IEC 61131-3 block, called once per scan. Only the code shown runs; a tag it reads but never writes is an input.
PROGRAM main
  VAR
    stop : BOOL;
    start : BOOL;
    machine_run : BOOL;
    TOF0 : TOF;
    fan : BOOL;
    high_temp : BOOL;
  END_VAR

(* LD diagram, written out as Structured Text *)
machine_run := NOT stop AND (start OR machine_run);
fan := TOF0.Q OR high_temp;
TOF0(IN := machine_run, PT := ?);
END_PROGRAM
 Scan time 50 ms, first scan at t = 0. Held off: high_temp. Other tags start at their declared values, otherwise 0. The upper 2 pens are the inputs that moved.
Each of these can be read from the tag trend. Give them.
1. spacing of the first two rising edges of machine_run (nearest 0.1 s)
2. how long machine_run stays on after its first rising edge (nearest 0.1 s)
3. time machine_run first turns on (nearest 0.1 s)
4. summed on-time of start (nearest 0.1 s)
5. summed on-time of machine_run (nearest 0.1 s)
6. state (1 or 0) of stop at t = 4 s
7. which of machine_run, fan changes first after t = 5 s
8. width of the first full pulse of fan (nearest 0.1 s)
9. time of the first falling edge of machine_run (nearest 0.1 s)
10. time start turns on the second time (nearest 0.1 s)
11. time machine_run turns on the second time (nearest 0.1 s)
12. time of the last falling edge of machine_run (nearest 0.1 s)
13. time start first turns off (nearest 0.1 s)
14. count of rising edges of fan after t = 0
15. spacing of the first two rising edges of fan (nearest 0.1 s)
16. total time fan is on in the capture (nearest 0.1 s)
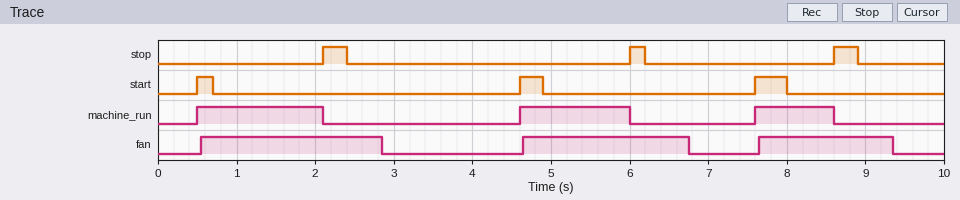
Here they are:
4.1 s
1.6 s
0.5 s
0.9 s
4.0 s
0
machine_run
2.3 s
2.1 s
4.6 s
4.6 s
8.6 s
0.7 s
3
4.1 s
6.1 s
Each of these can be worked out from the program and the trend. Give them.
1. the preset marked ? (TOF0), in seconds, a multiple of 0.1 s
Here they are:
0.7 s
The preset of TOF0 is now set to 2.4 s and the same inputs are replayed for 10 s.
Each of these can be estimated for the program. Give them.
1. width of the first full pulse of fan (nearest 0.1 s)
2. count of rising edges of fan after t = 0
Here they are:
4.0 s
2
